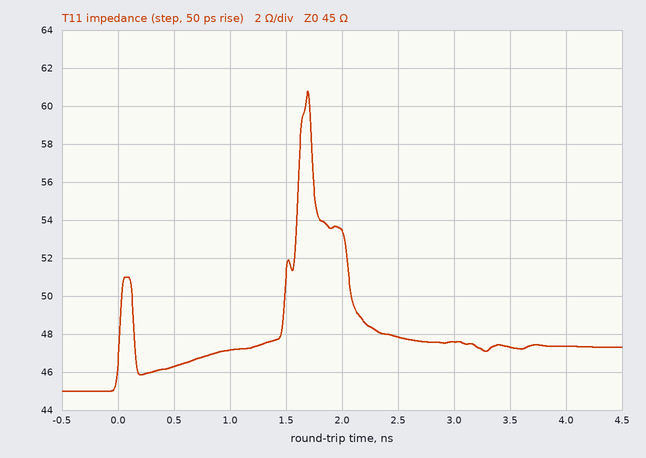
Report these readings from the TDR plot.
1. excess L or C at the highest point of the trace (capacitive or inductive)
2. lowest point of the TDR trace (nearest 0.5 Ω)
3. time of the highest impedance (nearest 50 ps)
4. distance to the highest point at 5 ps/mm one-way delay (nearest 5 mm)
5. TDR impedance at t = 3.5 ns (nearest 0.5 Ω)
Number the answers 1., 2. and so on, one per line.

1. inductive
2. 45.0 Ω
3. 1.70 ns
4. 170 mm
5. 47.5 Ω
